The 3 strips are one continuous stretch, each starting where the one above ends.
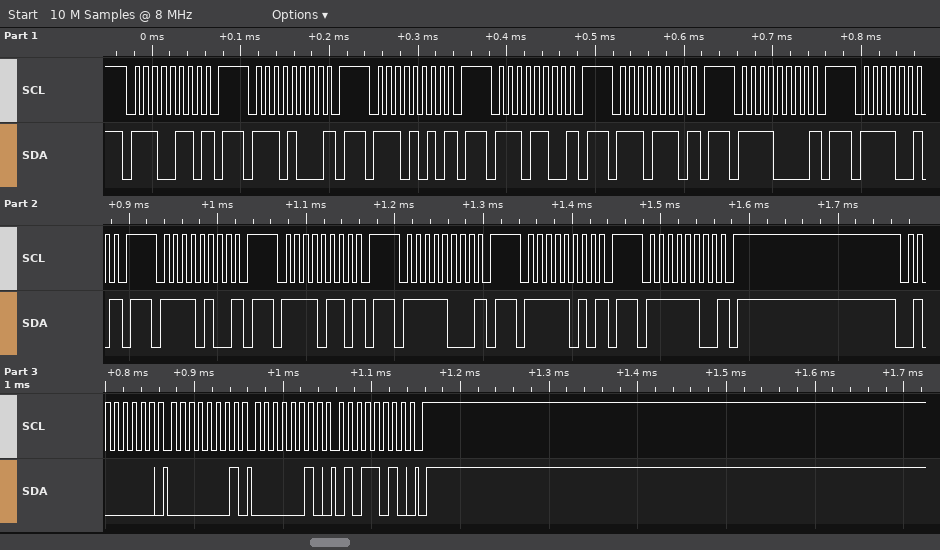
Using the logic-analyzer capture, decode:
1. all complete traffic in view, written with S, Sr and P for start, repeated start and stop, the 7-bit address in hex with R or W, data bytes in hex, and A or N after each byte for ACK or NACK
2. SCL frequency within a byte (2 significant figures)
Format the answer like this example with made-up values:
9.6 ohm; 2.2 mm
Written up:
S 73W N P S 74W N P S 75W N P S 76W N P S 77W N P S 78W N P S 79W N P S 7AW N P S 7BW N P S 7CW N P S 7DW N P S 7EW N P S 20W A 01 A 02 A 5A A P; 100 kHz
